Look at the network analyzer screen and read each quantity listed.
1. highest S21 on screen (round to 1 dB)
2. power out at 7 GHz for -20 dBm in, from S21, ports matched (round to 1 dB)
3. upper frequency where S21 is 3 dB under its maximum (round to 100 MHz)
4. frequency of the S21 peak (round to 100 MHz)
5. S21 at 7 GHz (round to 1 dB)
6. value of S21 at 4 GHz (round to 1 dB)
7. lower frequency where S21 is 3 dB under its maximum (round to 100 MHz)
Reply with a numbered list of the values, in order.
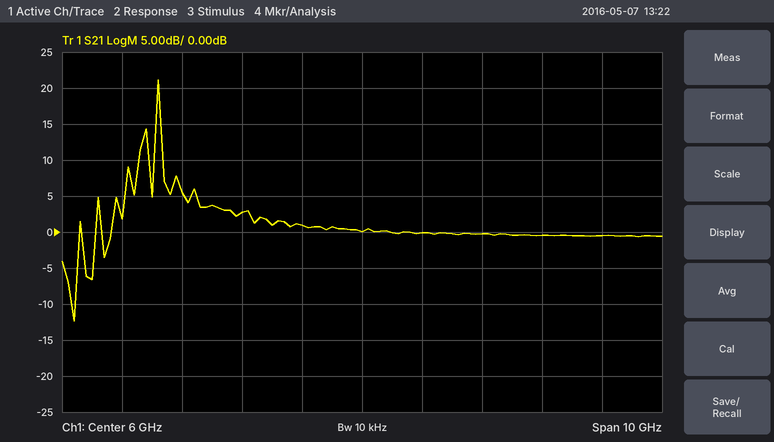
1. 21 dB
2. -20 dBm
3. 2.6 GHz
4. 2.6 GHz
5. 0 dB
6. 3 dB
7. 2.6 GHz
